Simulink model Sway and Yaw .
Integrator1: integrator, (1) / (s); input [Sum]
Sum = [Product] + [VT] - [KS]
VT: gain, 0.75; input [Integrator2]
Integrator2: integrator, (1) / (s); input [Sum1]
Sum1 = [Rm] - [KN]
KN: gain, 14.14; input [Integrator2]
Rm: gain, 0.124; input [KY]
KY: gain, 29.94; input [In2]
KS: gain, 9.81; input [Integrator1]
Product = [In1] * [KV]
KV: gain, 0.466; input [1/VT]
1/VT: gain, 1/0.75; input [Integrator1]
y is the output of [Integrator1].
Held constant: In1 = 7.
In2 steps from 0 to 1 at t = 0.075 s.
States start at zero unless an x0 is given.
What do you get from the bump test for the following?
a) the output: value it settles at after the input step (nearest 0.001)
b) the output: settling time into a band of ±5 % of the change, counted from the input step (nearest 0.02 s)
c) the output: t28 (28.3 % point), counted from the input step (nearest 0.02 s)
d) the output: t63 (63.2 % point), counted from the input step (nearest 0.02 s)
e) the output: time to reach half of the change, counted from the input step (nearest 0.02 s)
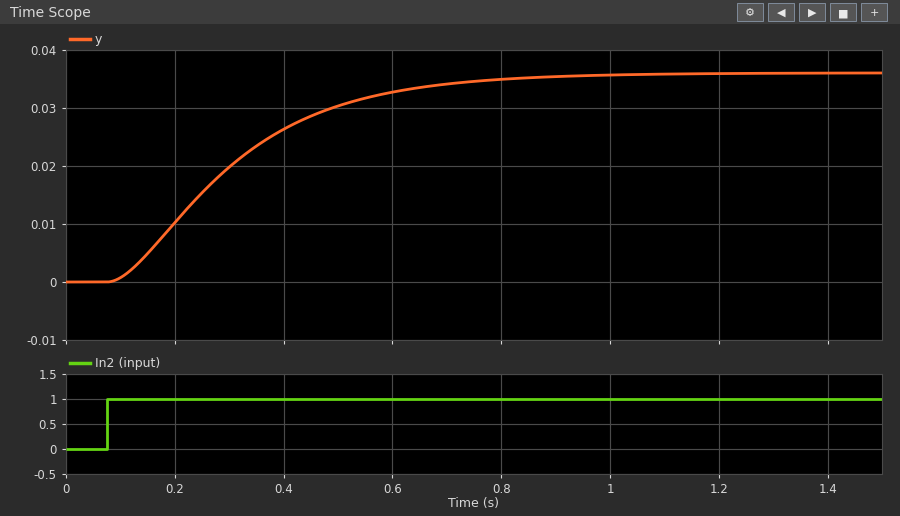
0.036
0.64 s
0.12 s
0.26 s
0.20 s
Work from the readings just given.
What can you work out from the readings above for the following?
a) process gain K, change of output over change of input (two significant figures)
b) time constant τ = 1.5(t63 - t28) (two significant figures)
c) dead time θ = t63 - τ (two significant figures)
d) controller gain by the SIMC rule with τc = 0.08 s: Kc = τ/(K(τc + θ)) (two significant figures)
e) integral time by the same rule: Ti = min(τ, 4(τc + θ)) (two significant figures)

0.036
0.21 s
0.050 s
45
0.21 s
